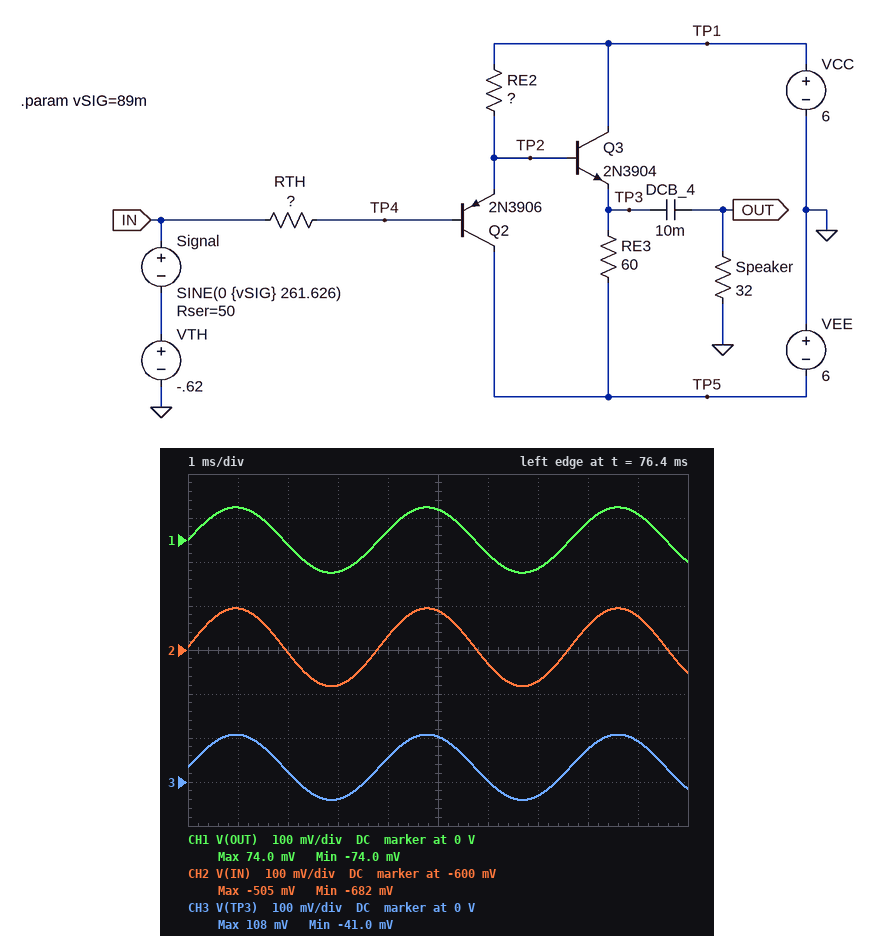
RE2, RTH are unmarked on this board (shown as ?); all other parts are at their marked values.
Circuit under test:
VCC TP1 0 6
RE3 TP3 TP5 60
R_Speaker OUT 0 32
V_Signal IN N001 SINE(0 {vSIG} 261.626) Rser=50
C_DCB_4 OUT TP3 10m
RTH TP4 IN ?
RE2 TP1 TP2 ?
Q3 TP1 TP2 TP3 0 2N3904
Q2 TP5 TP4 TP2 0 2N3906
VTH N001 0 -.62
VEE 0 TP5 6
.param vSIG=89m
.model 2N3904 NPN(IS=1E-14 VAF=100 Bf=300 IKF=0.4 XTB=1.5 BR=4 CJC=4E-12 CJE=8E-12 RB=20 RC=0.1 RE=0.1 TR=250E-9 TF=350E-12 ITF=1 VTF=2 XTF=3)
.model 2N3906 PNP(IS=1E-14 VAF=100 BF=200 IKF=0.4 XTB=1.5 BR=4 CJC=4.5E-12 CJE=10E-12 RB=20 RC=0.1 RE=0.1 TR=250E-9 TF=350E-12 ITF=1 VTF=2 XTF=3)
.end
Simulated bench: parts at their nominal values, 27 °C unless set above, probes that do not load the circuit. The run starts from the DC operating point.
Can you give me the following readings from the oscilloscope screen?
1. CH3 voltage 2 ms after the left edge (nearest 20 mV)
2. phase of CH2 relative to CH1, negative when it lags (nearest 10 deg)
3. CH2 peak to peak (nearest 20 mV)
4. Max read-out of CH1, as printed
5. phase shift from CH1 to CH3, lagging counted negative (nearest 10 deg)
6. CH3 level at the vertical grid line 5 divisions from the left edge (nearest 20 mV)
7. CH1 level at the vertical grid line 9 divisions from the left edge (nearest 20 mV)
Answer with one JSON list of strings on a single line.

["20 mV", "0 deg", "180 mV", "74.0 mV", "0 deg", "100 mV", "60 mV"]
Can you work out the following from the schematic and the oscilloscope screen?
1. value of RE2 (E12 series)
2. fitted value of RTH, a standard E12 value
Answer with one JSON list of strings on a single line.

["56 Ω", "1.2 kΩ"]
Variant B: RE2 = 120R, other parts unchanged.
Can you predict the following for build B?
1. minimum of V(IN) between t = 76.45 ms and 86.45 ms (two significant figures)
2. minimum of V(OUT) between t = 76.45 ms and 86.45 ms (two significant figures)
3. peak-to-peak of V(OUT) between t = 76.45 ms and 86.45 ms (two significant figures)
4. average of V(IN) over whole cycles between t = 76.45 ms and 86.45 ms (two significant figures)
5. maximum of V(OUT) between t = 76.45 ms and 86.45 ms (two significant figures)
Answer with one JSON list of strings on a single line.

["-700 mV", "-81 mV", "160 mV", "-610 mV", "81 mV"]
